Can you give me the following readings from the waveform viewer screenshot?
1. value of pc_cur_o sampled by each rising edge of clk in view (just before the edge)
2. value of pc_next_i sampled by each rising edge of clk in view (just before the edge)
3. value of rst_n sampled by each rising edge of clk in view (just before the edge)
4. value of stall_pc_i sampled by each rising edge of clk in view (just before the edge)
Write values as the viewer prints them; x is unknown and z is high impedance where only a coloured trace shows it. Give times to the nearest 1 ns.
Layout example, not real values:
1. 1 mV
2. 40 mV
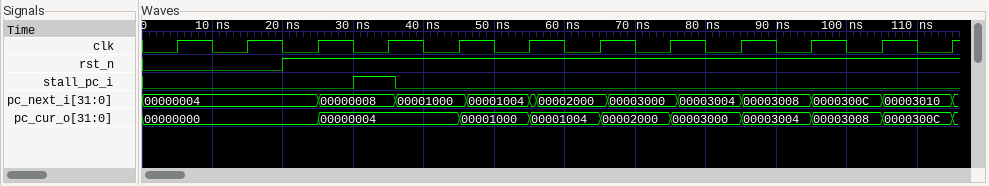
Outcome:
1. 00000000, 00000000, 00000000, 00000004, 00000004, 00001000, 00001004, 00002000, 00003000, 00003004, 00003008, 0000300C
2. 00000004, 00000004, 00000004, 00000008, 00001000, 00001004, 00002000, 00003000, 00003004, 00003008, 0000300C, 00003010
3. 0 0 1 1 1 1 1 1 1 1 1 1
4. 0 0 0 1 0 0 0 0 0 0 0 0
